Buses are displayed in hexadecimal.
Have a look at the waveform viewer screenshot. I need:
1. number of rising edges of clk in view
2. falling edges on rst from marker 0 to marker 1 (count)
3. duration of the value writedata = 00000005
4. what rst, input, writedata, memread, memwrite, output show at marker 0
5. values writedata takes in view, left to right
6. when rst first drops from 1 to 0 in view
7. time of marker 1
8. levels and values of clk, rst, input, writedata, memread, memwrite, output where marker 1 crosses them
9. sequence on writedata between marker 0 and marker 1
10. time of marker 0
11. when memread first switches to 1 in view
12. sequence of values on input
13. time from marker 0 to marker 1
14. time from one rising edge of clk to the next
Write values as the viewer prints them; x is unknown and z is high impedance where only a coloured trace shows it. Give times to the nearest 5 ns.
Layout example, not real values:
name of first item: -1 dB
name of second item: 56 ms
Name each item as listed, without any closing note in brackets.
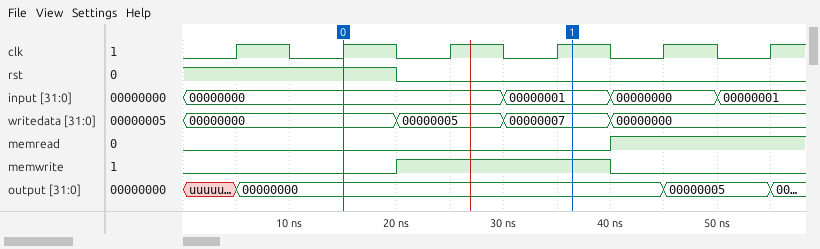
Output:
number of rising edges of clk in view: 6
falling edges on rst from marker 0 to marker 1: 1
duration of the value writedata = 00000005: 10 ns
what rst, input, writedata, memread, memwrite, output show at marker 0: rst=1, input=00000000, writedata=00000000, memread=0, memwrite=0, output=00000000
values writedata takes in view, left to right: 00000000, 00000005, 00000007, 00000000
when rst first drops from 1 to 0 in view: 20 ns
time of marker 1: 35 ns
levels and values of clk, rst, input, writedata, memread, memwrite, output where marker 1 crosses them: clk=1, rst=0, input=00000001, writedata=00000007, memread=0, memwrite=1, output=00000000
sequence on writedata between marker 0 and marker 1: 00000000, 00000005, 00000007
time of marker 0: 15 ns
when memread first switches to 1 in view: 40 ns
sequence of values on input: 00000000, 00000001, 00000000, 00000001
time from marker 0 to marker 1: 20 ns
time from one rising edge of clk to the next: 10 ns
